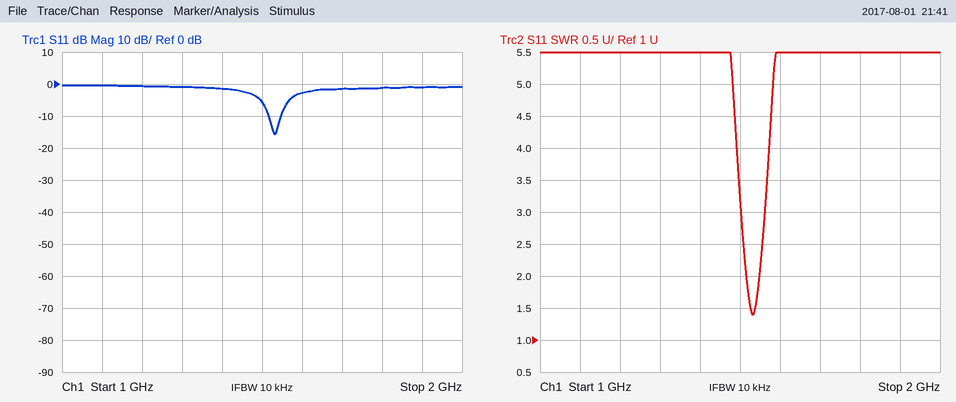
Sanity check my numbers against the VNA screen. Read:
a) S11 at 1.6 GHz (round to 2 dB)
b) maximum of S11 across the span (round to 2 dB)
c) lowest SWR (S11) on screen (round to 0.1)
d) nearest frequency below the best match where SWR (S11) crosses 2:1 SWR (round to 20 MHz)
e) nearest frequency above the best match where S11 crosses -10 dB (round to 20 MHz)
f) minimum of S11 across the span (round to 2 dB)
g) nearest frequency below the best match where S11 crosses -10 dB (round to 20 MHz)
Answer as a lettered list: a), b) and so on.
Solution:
a) -2 dB
b) 0 dB
c) 1.4
d) 1.52 GHz
e) 1.54 GHz
f) -16 dB
g) 1.52 GHz
